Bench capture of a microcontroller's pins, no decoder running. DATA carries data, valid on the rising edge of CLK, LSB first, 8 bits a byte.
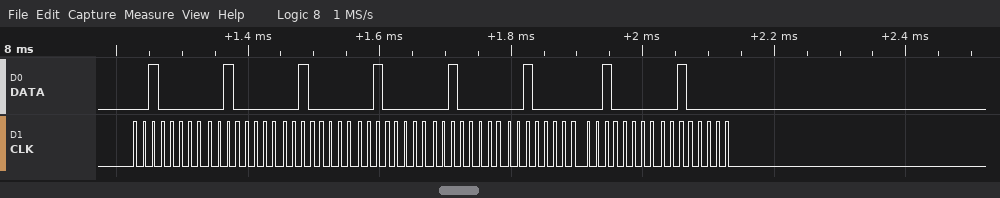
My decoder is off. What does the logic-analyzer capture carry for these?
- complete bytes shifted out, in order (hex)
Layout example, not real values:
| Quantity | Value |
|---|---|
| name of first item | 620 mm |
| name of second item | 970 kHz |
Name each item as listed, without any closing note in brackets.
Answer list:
| Quantity | Value |
|---|---|
| complete bytes shifted out, in order | 04 04 04 04 04 04 04 04 |
